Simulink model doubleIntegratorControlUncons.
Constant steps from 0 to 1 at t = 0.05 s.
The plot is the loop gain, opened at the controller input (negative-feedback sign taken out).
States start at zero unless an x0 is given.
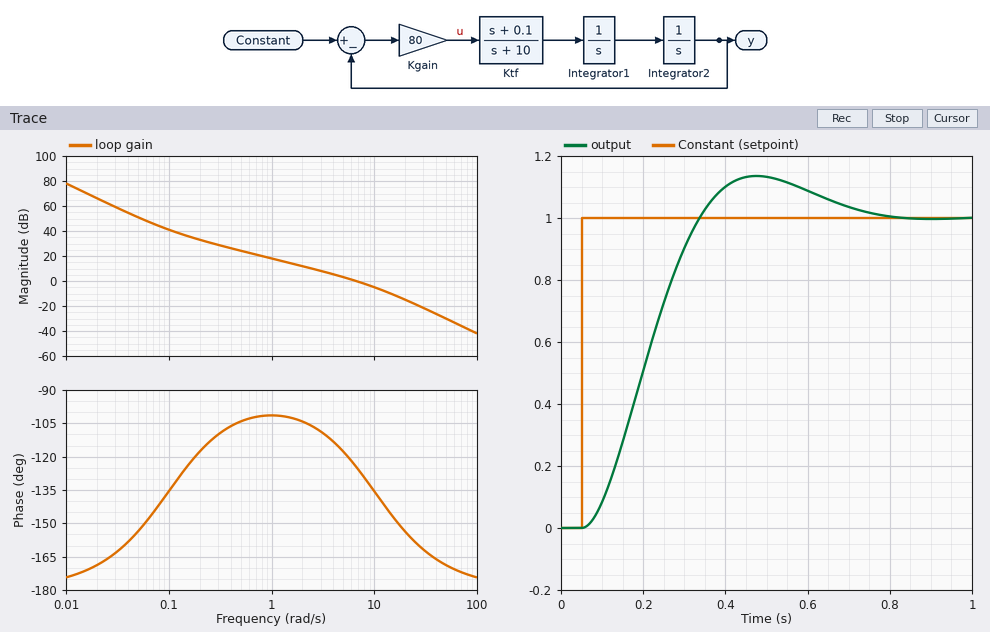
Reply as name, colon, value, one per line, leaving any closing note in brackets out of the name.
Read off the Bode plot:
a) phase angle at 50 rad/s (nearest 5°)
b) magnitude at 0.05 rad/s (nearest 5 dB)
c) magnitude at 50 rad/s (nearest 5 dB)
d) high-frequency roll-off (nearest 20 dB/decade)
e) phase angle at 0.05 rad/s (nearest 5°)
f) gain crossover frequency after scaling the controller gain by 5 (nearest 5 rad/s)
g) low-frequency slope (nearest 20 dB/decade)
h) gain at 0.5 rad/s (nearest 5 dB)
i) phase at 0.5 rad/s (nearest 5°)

phase angle at 50 rad/s: -170°
magnitude at 0.05 rad/s: 50 dB
magnitude at 50 rad/s: -30 dB
high-frequency roll-off: -40 dB/decade
phase angle at 0.05 rad/s: -155°
gain crossover frequency after scaling the controller gain by 5: 20 rad/s
low-frequency slope: -40 dB/decade
gain at 0.5 rad/s: 25 dB
phase at 0.5 rad/s: -105°
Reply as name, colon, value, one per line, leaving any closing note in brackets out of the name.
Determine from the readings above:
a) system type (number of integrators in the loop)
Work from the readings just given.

system type: 2
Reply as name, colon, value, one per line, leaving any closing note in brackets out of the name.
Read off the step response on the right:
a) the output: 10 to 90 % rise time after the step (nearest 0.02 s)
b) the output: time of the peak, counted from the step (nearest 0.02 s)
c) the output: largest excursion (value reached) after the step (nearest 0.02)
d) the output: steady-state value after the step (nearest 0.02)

the output: 10 to 90 % rise time after the step: 0.20 s
the output: time of the peak, counted from the step: 0.42 s
the output: largest excursion (value reached) after the step: 1.14
the output: steady-state value after the step: 1.00
